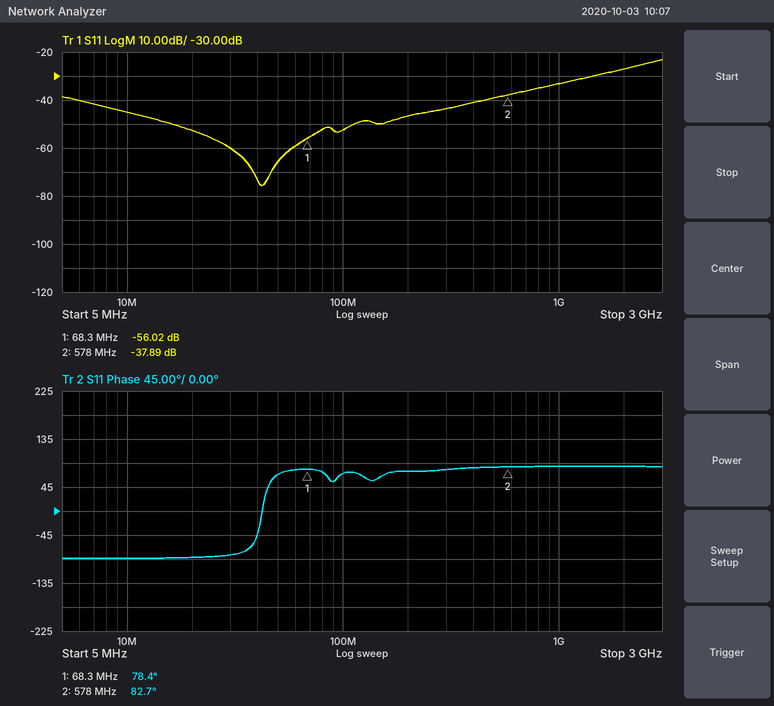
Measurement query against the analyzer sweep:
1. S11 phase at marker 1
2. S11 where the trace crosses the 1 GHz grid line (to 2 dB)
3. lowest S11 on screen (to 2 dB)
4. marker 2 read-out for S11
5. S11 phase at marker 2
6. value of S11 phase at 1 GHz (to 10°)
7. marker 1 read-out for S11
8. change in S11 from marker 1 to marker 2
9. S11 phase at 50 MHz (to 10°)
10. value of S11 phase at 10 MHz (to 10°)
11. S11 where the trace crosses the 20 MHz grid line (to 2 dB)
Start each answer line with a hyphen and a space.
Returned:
- 78.4°
- -34 dB
- -76 dB
- -37.89 dB
- 82.7°
- 80°
- -56.02 dB
- 18.13 dB
- 70°
- -90°
- -52 dB
